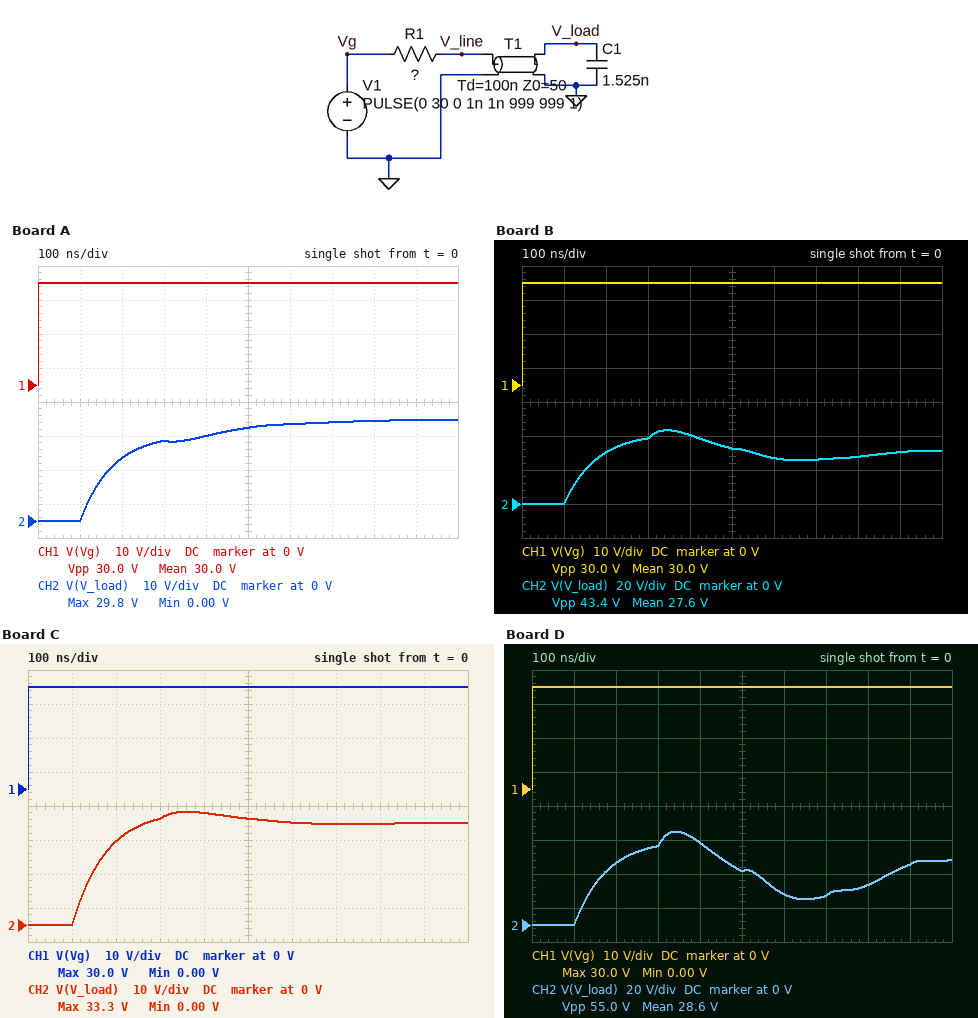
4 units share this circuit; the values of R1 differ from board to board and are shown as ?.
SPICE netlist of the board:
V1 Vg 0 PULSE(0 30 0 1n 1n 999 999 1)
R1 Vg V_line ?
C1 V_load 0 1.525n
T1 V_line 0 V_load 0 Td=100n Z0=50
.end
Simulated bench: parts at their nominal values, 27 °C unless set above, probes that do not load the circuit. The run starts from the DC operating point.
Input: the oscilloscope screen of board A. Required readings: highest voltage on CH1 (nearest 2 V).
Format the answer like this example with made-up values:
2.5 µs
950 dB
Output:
30 V
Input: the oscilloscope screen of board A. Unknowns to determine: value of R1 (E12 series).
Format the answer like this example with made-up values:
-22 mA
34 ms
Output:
68 Ω
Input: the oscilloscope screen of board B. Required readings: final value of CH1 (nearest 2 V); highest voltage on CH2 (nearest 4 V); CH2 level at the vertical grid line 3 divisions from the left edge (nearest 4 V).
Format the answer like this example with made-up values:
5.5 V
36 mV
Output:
30 V
44 V
40 V
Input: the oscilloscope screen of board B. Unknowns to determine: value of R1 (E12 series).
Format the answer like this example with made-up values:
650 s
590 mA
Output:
22 Ω
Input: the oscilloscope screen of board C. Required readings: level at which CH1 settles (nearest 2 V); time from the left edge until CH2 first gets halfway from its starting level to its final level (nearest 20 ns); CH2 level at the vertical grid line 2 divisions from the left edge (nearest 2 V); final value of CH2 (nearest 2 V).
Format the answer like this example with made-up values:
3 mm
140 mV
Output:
30 V
140 ns
24 V
30 V
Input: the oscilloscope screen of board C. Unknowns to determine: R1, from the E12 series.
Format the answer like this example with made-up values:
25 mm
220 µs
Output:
39 Ω
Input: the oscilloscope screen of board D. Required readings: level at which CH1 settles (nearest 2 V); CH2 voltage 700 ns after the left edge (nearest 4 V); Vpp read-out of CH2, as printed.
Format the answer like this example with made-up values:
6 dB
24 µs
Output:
30 V
16 V
55.0 V
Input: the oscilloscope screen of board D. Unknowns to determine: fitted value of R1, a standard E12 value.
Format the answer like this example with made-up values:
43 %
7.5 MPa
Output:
10 Ω
